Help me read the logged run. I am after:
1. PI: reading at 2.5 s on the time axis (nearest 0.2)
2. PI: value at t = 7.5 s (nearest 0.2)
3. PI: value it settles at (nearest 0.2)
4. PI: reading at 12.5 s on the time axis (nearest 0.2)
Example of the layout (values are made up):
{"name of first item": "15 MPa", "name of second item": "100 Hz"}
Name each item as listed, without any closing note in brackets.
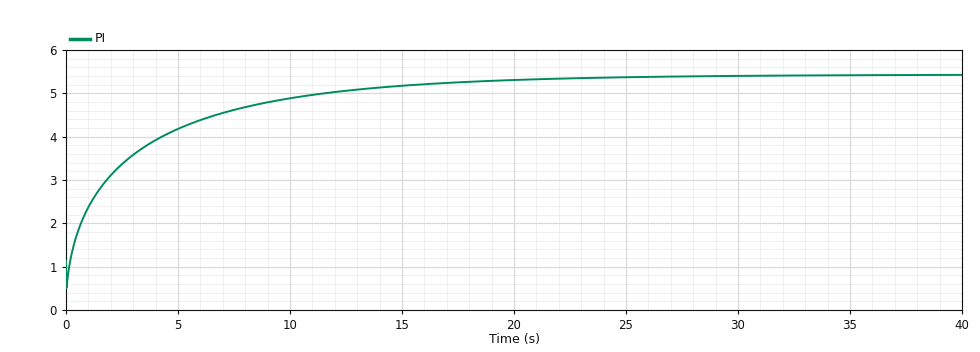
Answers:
{"PI: reading at 2.5 s on the time axis": "3.4", "PI: value at t = 7.5 s": "4.6", "PI: value it settles at": "5.4", "PI: reading at 12.5 s on the time axis": "5.0"}
